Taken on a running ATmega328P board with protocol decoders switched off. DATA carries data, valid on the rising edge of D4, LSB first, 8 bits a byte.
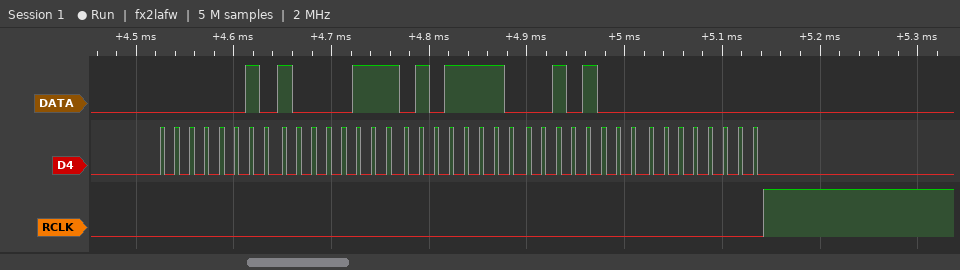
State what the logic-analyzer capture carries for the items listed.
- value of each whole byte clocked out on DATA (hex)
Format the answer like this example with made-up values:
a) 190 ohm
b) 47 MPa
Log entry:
a) 40 E1 7A 14 00
